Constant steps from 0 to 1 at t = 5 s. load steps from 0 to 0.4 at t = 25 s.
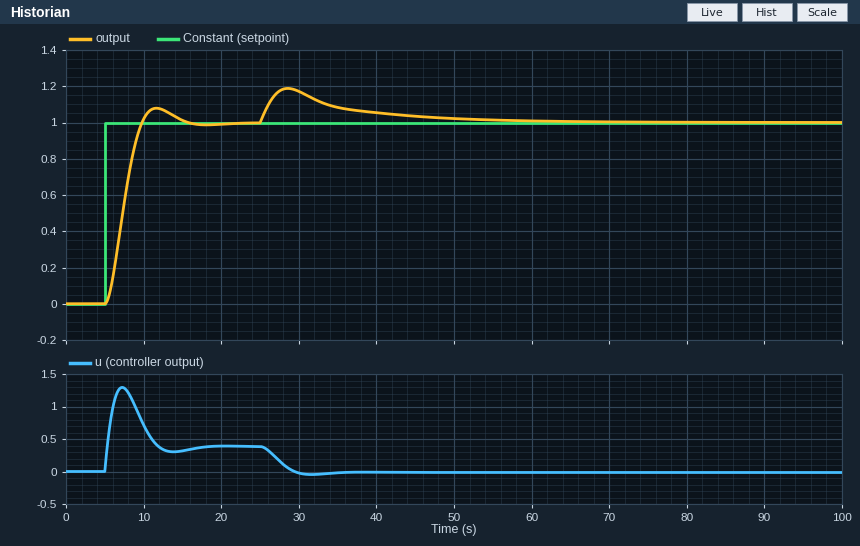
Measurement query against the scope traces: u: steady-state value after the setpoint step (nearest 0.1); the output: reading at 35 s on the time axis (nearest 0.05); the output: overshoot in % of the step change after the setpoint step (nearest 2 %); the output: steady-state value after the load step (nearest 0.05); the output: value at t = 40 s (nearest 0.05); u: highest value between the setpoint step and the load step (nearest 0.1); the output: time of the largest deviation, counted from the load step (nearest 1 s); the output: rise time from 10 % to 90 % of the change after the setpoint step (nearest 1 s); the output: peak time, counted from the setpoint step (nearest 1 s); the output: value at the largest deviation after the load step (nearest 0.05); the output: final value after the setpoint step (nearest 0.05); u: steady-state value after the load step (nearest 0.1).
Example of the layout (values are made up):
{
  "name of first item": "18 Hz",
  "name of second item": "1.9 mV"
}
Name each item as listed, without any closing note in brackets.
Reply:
{
  "u: steady-state value after the setpoint step": "0.4",
  "the output: reading at 35 s on the time axis": "1.10",
  "the output: overshoot in % of the step change after the setpoint step": "8 %",
  "the output: steady-state value after the load step": "1.00",
  "the output: value at t = 40 s": "1.05",
  "u: highest value between the setpoint step and the load step": "1.3",
  "the output: time of the largest deviation, counted from the load step": "4 s",
  "the output: rise time from 10 % to 90 % of the change after the setpoint step": "3 s",
  "the output: peak time, counted from the setpoint step": "7 s",
  "the output: value at the largest deviation after the load step": "1.20",
  "the output: final value after the setpoint step": "1.00",
  "u: steady-state value after the load step": "0.0"
}
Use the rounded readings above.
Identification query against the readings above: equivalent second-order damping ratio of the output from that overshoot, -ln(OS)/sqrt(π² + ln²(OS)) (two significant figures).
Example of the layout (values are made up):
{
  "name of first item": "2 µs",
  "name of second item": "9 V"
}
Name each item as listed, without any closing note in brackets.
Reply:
{
  "equivalent second-order damping ratio of the output from that overshoot, -ln(OS)/sqrt(π² + ln²(OS))": "0.63"
}
